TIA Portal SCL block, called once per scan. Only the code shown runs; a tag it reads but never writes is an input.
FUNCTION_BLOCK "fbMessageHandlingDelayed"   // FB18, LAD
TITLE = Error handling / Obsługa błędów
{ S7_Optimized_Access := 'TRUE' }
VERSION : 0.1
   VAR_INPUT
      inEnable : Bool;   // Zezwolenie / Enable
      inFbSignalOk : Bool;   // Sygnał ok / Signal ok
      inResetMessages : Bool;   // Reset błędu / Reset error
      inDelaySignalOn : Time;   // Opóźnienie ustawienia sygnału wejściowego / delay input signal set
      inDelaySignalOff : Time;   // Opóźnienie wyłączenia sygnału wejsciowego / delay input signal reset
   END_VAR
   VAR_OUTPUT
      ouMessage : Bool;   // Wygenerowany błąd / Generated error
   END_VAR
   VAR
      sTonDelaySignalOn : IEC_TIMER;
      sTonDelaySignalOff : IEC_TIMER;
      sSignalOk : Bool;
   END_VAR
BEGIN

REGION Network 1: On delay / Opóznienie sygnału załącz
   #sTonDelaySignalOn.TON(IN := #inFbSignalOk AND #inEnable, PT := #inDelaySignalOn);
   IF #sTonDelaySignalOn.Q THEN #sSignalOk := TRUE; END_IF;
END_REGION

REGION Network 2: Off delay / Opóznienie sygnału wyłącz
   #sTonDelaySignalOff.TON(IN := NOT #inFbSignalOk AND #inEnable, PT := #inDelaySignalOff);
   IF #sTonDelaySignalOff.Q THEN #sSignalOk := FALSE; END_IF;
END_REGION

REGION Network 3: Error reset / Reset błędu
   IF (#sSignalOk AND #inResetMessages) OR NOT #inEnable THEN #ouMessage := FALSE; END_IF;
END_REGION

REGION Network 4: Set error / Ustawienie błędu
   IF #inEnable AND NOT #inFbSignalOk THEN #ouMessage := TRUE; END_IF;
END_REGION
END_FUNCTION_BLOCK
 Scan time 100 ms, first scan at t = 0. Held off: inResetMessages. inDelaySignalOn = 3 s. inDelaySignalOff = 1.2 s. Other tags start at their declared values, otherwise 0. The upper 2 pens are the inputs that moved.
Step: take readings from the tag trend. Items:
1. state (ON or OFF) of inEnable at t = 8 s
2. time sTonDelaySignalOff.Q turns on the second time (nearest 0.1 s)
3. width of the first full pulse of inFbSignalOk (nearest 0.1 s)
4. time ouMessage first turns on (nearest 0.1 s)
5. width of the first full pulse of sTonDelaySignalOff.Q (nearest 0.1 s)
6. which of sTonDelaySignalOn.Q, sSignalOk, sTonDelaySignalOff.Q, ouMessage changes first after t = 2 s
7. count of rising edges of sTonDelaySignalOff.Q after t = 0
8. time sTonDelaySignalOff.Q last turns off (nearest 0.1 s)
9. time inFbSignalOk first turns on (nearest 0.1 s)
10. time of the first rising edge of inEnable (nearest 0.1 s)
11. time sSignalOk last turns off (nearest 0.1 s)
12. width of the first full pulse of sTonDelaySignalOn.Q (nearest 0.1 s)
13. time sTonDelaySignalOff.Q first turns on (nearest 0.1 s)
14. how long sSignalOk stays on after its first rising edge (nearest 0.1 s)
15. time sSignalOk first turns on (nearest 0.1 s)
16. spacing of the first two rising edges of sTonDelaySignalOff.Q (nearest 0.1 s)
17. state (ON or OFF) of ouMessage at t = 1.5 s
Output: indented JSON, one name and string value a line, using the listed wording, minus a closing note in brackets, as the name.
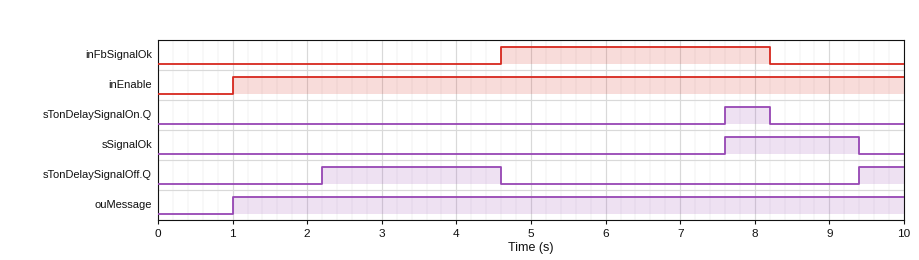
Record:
{
  "state (ON or OFF) of inEnable at t = 8 s": "ON",
  "time sTonDelaySignalOff.Q turns on the second time": "9.4 s",
  "width of the first full pulse of inFbSignalOk": "3.6 s",
  "time ouMessage first turns on": "1.0 s",
  "width of the first full pulse of sTonDelaySignalOff.Q": "2.4 s",
  "which of sTonDelaySignalOn.Q, sSignalOk, sTonDelaySignalOff.Q, ouMessage changes first after t = 2 s": "sTonDelaySignalOff.Q",
  "count of rising edges of sTonDelaySignalOff.Q after t = 0": "2",
  "time sTonDelaySignalOff.Q last turns off": "4.6 s",
  "time inFbSignalOk first turns on": "4.6 s",
  "time of the first rising edge of inEnable": "1.0 s",
  "time sSignalOk last turns off": "9.4 s",
  "width of the first full pulse of sTonDelaySignalOn.Q": "0.6 s",
  "time sTonDelaySignalOff.Q first turns on": "2.2 s",
  "how long sSignalOk stays on after its first rising edge": "1.8 s",
  "time sSignalOk first turns on": "7.6 s",
  "spacing of the first two rising edges of sTonDelaySignalOff.Q": "7.2 s",
  "state (ON or OFF) of ouMessage at t = 1.5 s": "ON"
}
